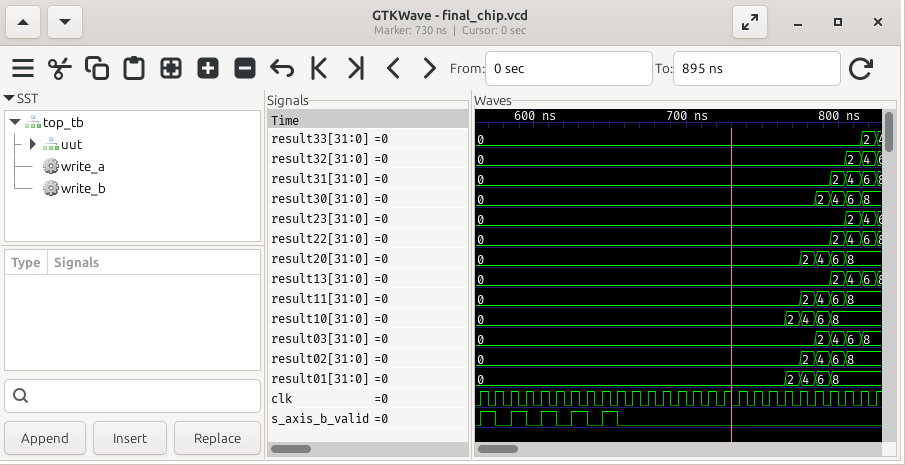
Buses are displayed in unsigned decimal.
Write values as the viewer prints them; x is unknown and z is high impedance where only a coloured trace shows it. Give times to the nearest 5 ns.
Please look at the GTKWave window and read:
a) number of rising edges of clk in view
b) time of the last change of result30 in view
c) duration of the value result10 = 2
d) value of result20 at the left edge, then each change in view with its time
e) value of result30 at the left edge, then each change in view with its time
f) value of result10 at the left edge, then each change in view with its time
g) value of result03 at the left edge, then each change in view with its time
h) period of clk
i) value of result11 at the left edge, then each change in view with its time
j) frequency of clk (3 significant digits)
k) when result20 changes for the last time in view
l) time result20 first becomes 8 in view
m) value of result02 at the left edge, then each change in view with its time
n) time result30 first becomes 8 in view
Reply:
27
815 ns
10 ns
0, 2 at 775 ns, 4 at 785 ns, 6 at 795 ns, 8 at 805 ns
0, 2 at 785 ns, 4 at 795 ns, 6 at 805 ns, 8 at 815 ns
0, 2 at 765 ns, 4 at 775 ns, 6 at 785 ns, 8 at 795 ns
0, 2 at 785 ns, 4 at 795 ns, 6 at 805 ns, 8 at 815 ns
10 ns
0, 2 at 775 ns, 4 at 785 ns, 6 at 795 ns, 8 at 805 ns
100 MHz
805 ns
805 ns
0, 2 at 775 ns, 4 at 785 ns, 6 at 795 ns, 8 at 805 ns
815 ns
